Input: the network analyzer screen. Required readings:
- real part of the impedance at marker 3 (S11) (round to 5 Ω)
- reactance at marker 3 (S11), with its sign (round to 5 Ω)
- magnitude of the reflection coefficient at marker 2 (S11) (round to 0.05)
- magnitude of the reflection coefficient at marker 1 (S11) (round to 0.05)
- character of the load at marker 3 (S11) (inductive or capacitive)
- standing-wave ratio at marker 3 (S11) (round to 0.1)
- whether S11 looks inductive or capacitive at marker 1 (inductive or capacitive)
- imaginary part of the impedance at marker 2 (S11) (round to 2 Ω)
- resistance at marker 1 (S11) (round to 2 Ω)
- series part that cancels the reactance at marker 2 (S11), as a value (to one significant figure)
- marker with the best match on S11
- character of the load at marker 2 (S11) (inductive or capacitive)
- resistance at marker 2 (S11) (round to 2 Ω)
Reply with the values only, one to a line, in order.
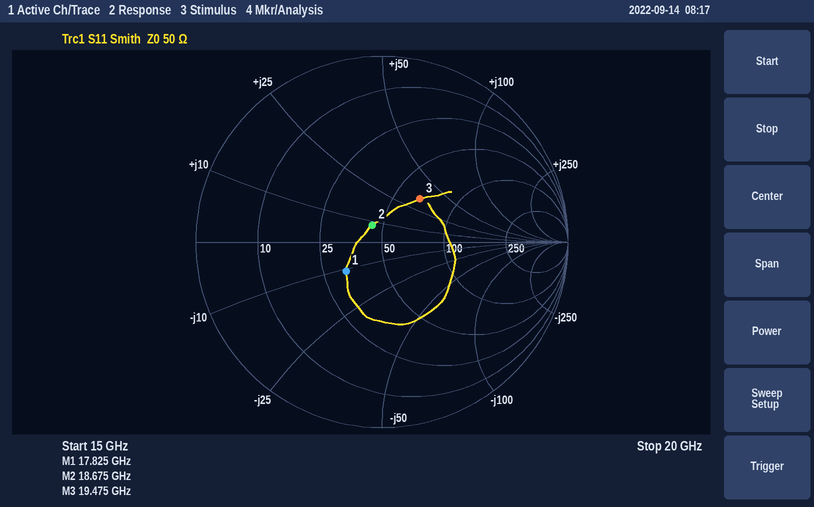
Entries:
65 Ω
+35 Ω
0.10
0.25
inductive
1.9
capacitive
+8 Ω
32 Ω
1 pF
marker 2
inductive
44 Ω
